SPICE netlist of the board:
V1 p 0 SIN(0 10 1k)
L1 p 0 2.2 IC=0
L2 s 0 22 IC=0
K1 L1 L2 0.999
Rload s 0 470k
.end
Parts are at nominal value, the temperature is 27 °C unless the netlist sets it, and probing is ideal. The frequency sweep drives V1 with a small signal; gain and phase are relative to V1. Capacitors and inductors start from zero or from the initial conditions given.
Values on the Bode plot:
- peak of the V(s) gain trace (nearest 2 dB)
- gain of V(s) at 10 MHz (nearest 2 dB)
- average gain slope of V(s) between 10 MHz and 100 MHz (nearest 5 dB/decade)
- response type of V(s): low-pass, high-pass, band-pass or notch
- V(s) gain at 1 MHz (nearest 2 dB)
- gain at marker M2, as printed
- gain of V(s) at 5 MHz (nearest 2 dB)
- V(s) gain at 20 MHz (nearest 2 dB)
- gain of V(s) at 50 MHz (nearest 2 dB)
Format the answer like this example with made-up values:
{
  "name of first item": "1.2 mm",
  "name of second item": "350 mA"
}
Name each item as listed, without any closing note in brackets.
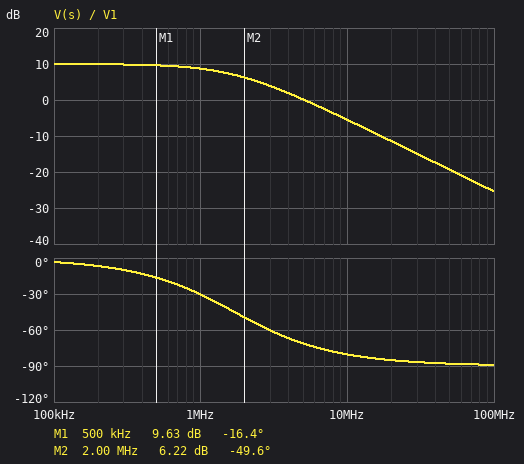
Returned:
{
  "peak of the V(s) gain trace": "10 dB",
  "gain of V(s) at 10 MHz": "-6 dB",
  "average gain slope of V(s) between 10 MHz and 100 MHz": "-20 dB/decade",
  "response type of V(s): low-pass, high-pass, band-pass or notch": "low-pass",
  "V(s) gain at 1 MHz": "8 dB",
  "gain at marker M2, as printed": "6.22 dB",
  "gain of V(s) at 5 MHz": "0 dB",
  "V(s) gain at 20 MHz": "-12 dB",
  "gain of V(s) at 50 MHz": "-20 dB"
}
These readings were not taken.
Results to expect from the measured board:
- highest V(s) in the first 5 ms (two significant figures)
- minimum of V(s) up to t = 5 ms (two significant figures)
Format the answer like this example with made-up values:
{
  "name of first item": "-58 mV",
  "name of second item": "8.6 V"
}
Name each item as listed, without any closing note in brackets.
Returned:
{
  "highest V(s) in the first 5 ms": "32 V",
  "minimum of V(s) up to t = 5 ms": "-32 V"
}
